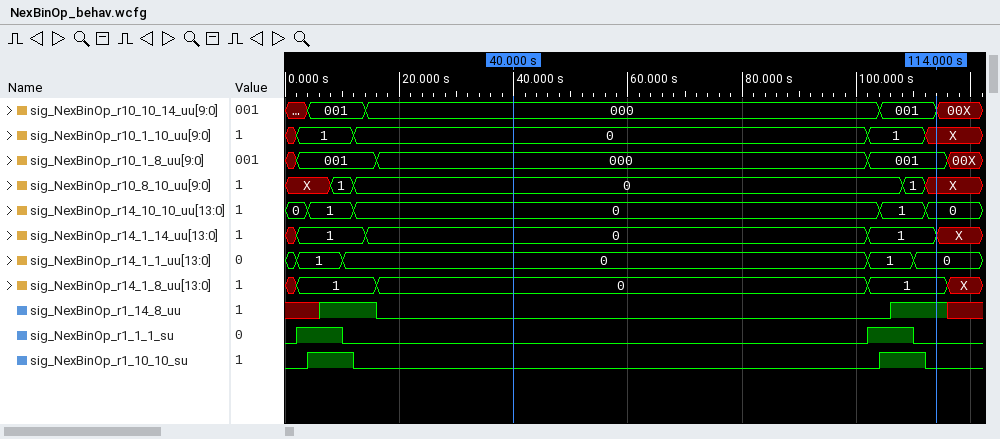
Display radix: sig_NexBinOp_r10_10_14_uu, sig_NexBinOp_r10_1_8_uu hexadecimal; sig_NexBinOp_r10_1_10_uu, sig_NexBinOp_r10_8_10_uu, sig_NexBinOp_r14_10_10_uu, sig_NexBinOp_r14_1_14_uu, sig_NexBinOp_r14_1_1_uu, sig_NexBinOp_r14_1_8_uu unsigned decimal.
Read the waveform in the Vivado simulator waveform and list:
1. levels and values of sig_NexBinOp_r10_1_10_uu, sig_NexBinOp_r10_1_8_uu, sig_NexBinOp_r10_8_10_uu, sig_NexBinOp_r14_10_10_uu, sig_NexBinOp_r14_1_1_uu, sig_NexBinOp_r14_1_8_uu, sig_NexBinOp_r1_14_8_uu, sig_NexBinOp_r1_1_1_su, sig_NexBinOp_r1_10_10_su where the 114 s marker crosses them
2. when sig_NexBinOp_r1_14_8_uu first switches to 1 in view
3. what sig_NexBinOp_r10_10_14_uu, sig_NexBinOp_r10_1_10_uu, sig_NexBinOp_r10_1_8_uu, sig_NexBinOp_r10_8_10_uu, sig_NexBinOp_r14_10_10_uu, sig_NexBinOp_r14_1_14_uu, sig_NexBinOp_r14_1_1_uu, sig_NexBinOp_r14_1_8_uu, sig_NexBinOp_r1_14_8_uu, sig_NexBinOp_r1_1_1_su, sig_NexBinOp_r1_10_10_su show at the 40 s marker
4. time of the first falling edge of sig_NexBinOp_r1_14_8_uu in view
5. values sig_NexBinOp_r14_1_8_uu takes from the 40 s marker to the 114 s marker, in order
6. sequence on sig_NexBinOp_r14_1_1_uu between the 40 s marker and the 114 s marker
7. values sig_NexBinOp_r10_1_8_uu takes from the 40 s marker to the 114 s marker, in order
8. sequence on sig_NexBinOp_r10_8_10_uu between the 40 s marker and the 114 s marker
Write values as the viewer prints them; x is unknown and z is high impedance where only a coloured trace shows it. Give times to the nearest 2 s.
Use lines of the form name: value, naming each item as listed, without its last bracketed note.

levels and values of sig_NexBinOp_r10_1_10_uu, sig_NexBinOp_r10_1_8_uu, sig_NexBinOp_r10_8_10_uu, sig_NexBinOp_r14_10_10_uu, sig_NexBinOp_r14_1_1_uu, sig_NexBinOp_r14_1_8_uu, sig_NexBinOp_r1_14_8_uu, sig_NexBinOp_r1_1_1_su, sig_NexBinOp_r1_10_10_su where the 114 s marker crosses them: sig_NexBinOp_r10_1_10_uu=X, sig_NexBinOp_r10_1_8_uu=001, sig_NexBinOp_r10_8_10_uu=X, sig_NexBinOp_r14_10_10_uu=0, sig_NexBinOp_r14_1_1_uu=0, sig_NexBinOp_r14_1_8_uu=1, sig_NexBinOp_r1_14_8_uu=1, sig_NexBinOp_r1_1_1_su=0, sig_NexBinOp_r1_10_10_su=0
when sig_NexBinOp_r1_14_8_uu first switches to 1 in view: 6 s
what sig_NexBinOp_r10_10_14_uu, sig_NexBinOp_r10_1_10_uu, sig_NexBinOp_r10_1_8_uu, sig_NexBinOp_r10_8_10_uu, sig_NexBinOp_r14_10_10_uu, sig_NexBinOp_r14_1_14_uu, sig_NexBinOp_r14_1_1_uu, sig_NexBinOp_r14_1_8_uu, sig_NexBinOp_r1_14_8_uu, sig_NexBinOp_r1_1_1_su, sig_NexBinOp_r1_10_10_su show at the 40 s marker: sig_NexBinOp_r10_10_14_uu=000, sig_NexBinOp_r10_1_10_uu=0, sig_NexBinOp_r10_1_8_uu=000, sig_NexBinOp_r10_8_10_uu=0, sig_NexBinOp_r14_10_10_uu=0, sig_NexBinOp_r14_1_14_uu=0, sig_NexBinOp_r14_1_1_uu=0, sig_NexBinOp_r14_1_8_uu=0, sig_NexBinOp_r1_14_8_uu=0, sig_NexBinOp_r1_1_1_su=0, sig_NexBinOp_r1_10_10_su=0
time of the first falling edge of sig_NexBinOp_r1_14_8_uu in view: 16 s
values sig_NexBinOp_r14_1_8_uu takes from the 40 s marker to the 114 s marker, in order: 0, 1
sequence on sig_NexBinOp_r14_1_1_uu between the 40 s marker and the 114 s marker: 0, 1, 0
values sig_NexBinOp_r10_1_8_uu takes from the 40 s marker to the 114 s marker, in order: 000, 001
sequence on sig_NexBinOp_r10_8_10_uu between the 40 s marker and the 114 s marker: 0, 1, X
